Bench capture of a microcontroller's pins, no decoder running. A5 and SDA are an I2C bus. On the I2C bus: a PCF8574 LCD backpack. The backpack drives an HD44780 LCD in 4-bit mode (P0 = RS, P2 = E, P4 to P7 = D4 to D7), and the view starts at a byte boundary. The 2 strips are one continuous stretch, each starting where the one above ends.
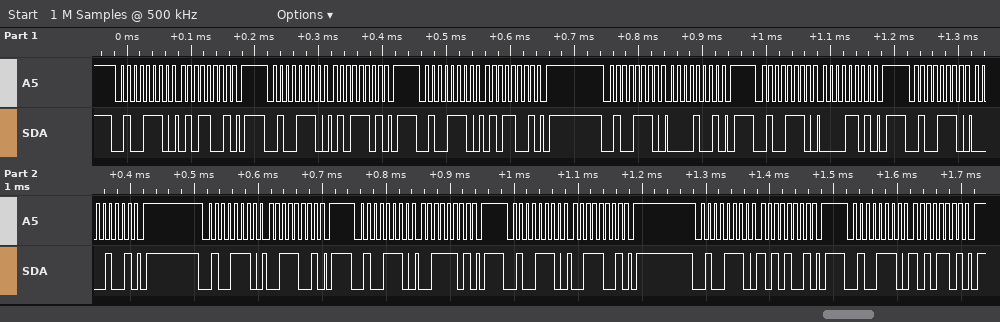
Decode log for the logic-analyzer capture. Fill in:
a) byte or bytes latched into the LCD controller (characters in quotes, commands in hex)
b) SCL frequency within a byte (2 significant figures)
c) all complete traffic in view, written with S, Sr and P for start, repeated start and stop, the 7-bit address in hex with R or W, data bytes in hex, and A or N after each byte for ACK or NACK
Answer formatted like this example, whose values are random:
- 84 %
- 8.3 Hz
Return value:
- 'P'
- 100 kHz
- S 27W A 59 A P S 27W A 5D A P S 27W A 59 A P S 27W A 09 A P S 27W A 0D A P S 27W A 09 A P S 27W A 39 A P S 27W A 3D A P S 27W A 39 A P S 27W A A9 A P S 27W A AD A P
